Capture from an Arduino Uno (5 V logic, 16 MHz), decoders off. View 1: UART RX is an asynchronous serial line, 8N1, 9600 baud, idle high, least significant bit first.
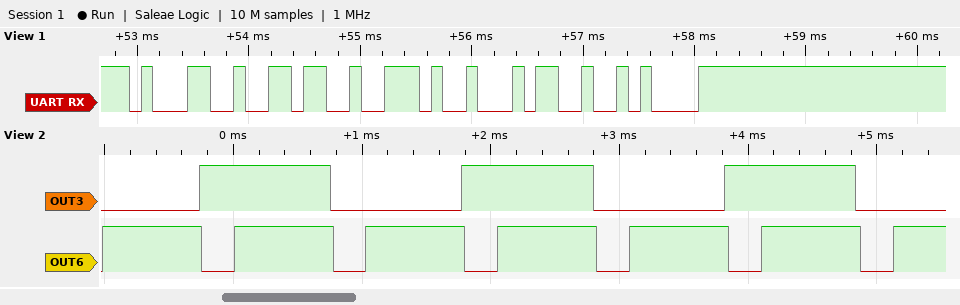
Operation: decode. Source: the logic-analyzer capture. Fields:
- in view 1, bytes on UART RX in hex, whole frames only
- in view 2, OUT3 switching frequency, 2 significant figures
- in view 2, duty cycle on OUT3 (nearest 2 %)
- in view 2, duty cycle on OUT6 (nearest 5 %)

31 36 2E 34 0A
490 Hz
50 %
75 %
